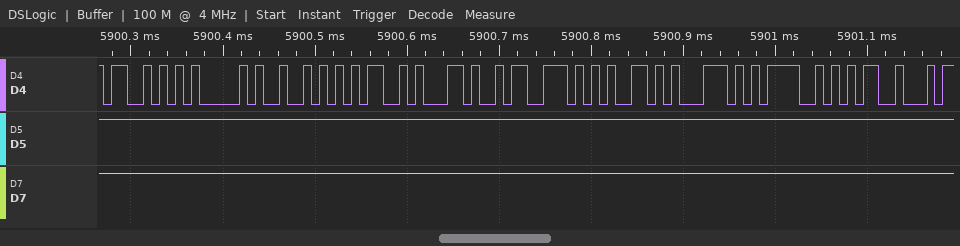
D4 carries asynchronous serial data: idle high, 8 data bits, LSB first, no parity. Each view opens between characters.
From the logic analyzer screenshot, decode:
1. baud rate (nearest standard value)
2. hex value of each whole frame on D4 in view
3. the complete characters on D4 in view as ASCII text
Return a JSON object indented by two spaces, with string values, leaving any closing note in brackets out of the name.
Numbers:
{
  "baud rate": "115200 baud",
  "hex value of each whole frame on D4 in view": "53, 41, 52, 4D, 2C, 73, 65, 71, 3D, 35",
  "the complete characters on D4 in view as ASCII text": "\"SARM,seq=5\""
}
